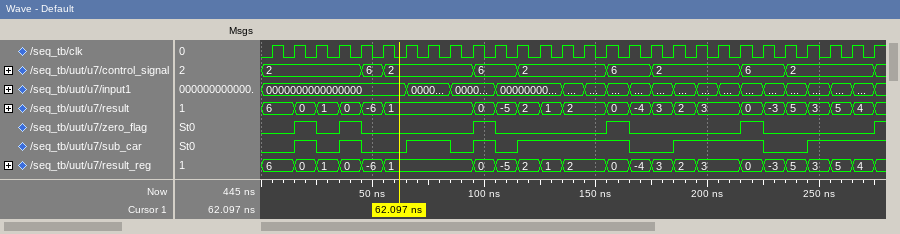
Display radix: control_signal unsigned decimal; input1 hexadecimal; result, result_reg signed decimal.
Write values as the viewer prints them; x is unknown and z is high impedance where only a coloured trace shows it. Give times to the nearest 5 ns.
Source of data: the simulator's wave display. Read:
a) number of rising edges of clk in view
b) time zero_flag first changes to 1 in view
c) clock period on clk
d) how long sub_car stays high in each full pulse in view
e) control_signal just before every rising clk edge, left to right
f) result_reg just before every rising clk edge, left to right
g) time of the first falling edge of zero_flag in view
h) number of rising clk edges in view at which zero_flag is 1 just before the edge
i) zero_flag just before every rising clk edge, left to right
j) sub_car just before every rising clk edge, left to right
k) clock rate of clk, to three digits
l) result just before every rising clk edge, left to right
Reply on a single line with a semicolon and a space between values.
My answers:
28; 15 ns; 10 ns; 10 ns, 10 ns, 20 ns, 10 ns, 50 ns, 40 ns; 2, 2, 2, 2, 2, 6, 2, 2, 2, 2, 6, 6, 2, 2, 2, 2, 6, 6, 2, 2, 2, 2, 6, 6, 2, 2, 2, 2; 6, 6, 0, 1, 0, -6, 1, 1, 1, 1, 0, -5, 2, 1, 2, 2, 0, -4, 3, 2, 3, 3, 0, -3, 5, 3, 5, 4; 25 ns; 5; 0 0 1 0 1 0 0 0 0 0 1 0 0 0 0 0 1 0 0 0 0 0 1 0 0 0 0 0; 0 0 1 0 1 0 0 1 1 0 1 0 1 1 1 1 1 0 0 1 1 1 1 0 0 1 1 1; 100 MHz; 6, 6, 0, 1, 0, -6, 1, 1, 1, 1, 0, -5, 2, 1, 2, 2, 0, -4, 3, 2, 3, 3, 0, -3, 5, 3, 5, 4
